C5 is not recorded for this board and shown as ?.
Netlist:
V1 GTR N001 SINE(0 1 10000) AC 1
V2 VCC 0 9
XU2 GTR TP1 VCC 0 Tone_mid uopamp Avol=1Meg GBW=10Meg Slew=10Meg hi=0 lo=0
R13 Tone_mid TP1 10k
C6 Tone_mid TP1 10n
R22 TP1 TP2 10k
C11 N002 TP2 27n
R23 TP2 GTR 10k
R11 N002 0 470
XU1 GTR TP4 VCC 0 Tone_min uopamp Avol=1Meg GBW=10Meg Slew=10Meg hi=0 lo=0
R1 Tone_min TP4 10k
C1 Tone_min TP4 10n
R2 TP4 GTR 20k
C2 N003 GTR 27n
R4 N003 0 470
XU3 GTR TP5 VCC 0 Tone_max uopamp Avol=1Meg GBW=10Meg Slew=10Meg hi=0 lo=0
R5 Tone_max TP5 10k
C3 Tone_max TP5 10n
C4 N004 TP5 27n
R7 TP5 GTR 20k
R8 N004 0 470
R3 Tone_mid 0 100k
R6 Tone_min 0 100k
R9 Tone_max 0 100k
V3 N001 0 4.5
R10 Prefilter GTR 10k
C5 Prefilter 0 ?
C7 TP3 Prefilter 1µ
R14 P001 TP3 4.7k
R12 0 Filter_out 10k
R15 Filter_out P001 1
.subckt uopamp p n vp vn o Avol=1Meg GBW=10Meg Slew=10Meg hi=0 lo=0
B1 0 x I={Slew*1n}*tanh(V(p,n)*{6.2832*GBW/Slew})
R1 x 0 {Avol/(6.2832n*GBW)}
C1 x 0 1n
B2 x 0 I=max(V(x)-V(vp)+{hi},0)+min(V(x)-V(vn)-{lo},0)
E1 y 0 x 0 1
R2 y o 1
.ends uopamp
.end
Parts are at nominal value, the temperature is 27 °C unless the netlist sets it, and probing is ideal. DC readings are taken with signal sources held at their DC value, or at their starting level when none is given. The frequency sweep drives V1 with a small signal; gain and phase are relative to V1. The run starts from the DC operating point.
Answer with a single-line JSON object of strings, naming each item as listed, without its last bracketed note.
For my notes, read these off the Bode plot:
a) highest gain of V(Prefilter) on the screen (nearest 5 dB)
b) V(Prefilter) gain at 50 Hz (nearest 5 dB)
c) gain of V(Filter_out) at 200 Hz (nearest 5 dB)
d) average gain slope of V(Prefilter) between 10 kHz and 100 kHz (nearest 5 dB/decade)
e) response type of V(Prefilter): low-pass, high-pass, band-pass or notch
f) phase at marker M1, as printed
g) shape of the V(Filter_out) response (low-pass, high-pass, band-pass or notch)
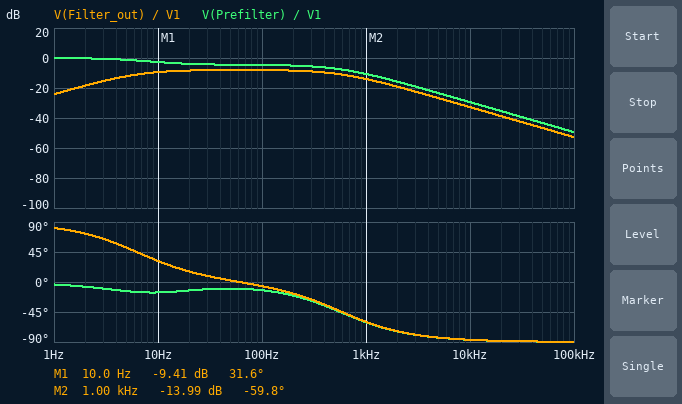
{"highest gain of V(Prefilter) on the screen": "0 dB", "V(Prefilter) gain at 50 Hz": "-5 dB", "gain of V(Filter_out) at 200 Hz": "-10 dB", "average gain slope of V(Prefilter) between 10 kHz and 100 kHz": "-20 dB/decade", "response type of V(Prefilter): low-pass, high-pass, band-pass or notch": "low-pass", "phase at marker M1, as printed": "31.6 deg", "shape of the V(Filter_out) response": "band-pass"}
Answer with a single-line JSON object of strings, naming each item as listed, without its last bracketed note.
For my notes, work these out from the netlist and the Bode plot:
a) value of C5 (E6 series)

{"value of C5": "47 nF"}
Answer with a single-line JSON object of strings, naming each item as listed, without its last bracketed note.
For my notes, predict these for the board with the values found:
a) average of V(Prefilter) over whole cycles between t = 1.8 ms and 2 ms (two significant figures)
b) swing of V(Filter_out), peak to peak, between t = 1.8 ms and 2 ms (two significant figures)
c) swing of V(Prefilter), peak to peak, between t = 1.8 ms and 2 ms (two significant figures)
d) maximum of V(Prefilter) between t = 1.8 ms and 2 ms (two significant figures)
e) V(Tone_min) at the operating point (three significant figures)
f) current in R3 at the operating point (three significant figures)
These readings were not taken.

{"average of V(Prefilter) over whole cycles between t = 1.8 ms and 2 ms": "4.5 V", "swing of V(Filter_out), peak to peak, between t = 1.8 ms and 2 ms": "46 mV", "swing of V(Prefilter), peak to peak, between t = 1.8 ms and 2 ms": "68 mV", "maximum of V(Prefilter) between t = 1.8 ms and 2 ms": "4.5 V", "V(Tone_min) at the operating point": "4.50 V", "current in R3 at the operating point": "45.0 µA"}
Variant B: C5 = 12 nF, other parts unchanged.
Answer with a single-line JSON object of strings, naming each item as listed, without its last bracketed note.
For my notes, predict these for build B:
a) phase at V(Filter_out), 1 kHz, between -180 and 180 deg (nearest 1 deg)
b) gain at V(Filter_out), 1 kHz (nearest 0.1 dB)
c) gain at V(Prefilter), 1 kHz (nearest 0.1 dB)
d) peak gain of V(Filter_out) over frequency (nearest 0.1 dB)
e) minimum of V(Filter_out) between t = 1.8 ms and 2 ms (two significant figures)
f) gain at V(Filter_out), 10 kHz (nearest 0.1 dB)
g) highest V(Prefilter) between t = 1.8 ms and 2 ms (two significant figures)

{"phase at V(Filter_out), 1 kHz, between -180 and 180 deg": "-24 deg", "gain at V(Filter_out), 1 kHz": "-8.7 dB", "gain at V(Prefilter), 1 kHz": "-5.3 dB", "peak gain of V(Filter_out) over frequency": "-7.9 dB", "minimum of V(Filter_out) between t = 1.8 ms and 2 ms": "-88 mV", "gain at V(Filter_out), 10 kHz": "-21.1 dB", "highest V(Prefilter) between t = 1.8 ms and 2 ms": "4.6 V"}
